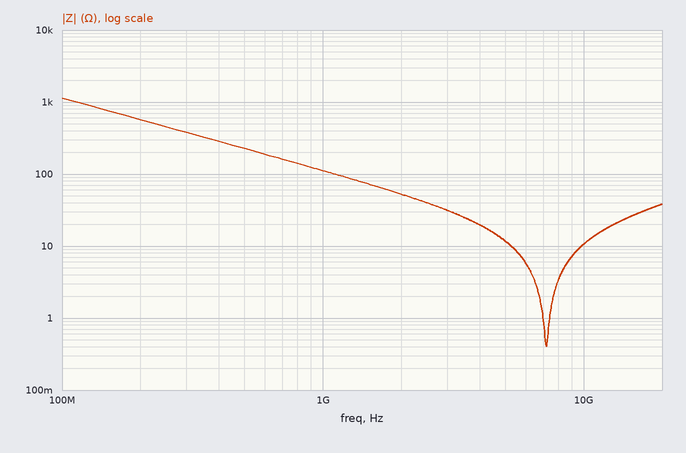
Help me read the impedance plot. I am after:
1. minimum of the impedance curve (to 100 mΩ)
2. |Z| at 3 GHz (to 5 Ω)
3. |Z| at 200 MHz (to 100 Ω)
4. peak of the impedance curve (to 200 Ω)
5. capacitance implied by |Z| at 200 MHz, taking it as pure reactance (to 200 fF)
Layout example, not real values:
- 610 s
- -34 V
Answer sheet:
- 400 mΩ
- 30 Ω
- 600 Ω
- 1.2 kΩ
- 1.4 pF
